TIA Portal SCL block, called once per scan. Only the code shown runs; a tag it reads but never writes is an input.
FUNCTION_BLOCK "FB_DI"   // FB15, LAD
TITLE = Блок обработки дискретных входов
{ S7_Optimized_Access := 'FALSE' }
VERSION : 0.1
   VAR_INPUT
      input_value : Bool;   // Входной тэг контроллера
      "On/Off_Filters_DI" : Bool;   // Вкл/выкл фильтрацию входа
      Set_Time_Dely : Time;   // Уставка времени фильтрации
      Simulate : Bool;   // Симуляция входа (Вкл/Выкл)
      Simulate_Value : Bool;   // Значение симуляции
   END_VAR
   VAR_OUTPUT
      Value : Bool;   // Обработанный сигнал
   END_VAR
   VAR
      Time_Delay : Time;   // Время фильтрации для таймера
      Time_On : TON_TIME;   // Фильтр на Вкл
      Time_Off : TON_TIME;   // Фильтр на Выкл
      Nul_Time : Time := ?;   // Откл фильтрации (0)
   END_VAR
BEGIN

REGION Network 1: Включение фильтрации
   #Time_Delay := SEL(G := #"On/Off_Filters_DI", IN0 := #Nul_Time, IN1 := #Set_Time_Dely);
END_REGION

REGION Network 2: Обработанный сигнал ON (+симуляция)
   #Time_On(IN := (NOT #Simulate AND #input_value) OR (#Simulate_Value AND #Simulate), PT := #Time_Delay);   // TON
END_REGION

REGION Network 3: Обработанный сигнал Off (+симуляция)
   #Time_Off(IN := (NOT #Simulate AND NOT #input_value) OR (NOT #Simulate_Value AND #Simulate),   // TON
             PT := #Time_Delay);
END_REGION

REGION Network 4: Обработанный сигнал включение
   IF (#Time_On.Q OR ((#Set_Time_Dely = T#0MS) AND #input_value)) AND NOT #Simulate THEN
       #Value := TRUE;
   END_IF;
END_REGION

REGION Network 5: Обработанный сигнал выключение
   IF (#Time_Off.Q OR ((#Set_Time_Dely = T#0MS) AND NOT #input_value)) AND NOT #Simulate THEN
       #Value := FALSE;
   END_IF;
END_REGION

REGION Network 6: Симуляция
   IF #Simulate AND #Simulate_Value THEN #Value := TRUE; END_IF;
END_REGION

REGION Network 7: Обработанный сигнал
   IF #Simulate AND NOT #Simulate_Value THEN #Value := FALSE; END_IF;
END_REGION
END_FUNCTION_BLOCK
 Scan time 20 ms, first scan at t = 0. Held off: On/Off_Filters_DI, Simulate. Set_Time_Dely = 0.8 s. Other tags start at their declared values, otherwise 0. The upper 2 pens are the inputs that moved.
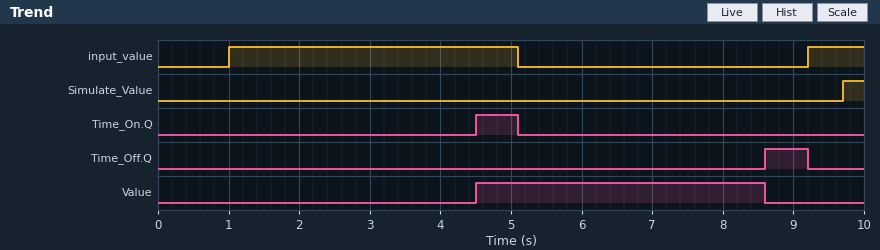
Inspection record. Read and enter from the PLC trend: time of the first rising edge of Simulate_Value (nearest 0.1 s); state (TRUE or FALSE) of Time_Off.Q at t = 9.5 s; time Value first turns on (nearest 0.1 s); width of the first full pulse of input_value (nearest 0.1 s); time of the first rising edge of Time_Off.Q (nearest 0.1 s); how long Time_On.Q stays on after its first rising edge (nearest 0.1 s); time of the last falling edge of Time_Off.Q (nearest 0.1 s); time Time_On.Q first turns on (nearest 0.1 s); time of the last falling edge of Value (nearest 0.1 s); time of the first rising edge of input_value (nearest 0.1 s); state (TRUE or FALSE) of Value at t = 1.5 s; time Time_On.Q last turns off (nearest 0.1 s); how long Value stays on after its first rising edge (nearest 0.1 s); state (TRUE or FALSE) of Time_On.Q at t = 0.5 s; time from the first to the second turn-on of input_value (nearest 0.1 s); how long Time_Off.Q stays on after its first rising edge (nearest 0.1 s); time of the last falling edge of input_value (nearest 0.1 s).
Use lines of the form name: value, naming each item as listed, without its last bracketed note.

time of the first rising edge of Simulate_Value: 9.7 s
state (TRUE or FALSE) of Time_Off.Q at t = 9.5 s: FALSE
time Value first turns on: 4.5 s
width of the first full pulse of input_value: 4.1 s
time of the first rising edge of Time_Off.Q: 8.6 s
how long Time_On.Q stays on after its first rising edge: 0.6 s
time of the last falling edge of Time_Off.Q: 9.2 s
time Time_On.Q first turns on: 4.5 s
time of the last falling edge of Value: 8.6 s
time of the first rising edge of input_value: 1.0 s
state (TRUE or FALSE) of Value at t = 1.5 s: FALSE
time Time_On.Q last turns off: 5.1 s
how long Value stays on after its first rising edge: 4.1 s
state (TRUE or FALSE) of Time_On.Q at t = 0.5 s: FALSE
time from the first to the second turn-on of input_value: 8.2 s
how long Time_Off.Q stays on after its first rising edge: 0.6 s
time of the last falling edge of input_value: 5.1 s
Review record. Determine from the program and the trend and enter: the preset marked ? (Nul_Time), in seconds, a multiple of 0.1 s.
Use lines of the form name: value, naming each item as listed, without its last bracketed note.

the preset marked ? (Nul_Time), in seconds, a multiple of 0.1 s: 3.5 s
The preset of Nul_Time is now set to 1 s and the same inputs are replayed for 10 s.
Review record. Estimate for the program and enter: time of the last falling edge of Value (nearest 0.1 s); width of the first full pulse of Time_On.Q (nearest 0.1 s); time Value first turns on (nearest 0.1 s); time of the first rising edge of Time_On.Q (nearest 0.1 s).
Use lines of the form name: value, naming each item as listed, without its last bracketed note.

time of the last falling edge of Value: 6.1 s
width of the first full pulse of Time_On.Q: 3.1 s
time Value first turns on: 2.0 s
time of the first rising edge of Time_On.Q: 2.0 s
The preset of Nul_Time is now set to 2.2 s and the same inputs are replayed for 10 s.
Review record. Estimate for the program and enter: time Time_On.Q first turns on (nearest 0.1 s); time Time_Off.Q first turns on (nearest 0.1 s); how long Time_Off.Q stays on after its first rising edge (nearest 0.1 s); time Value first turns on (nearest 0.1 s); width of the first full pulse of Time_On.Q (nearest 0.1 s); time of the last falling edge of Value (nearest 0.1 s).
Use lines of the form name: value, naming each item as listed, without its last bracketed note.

time Time_On.Q first turns on: 3.2 s
time Time_Off.Q first turns on: 7.3 s
how long Time_Off.Q stays on after its first rising edge: 1.9 s
time Value first turns on: 3.2 s
width of the first full pulse of Time_On.Q: 1.9 s
time of the last falling edge of Value: 7.3 s
